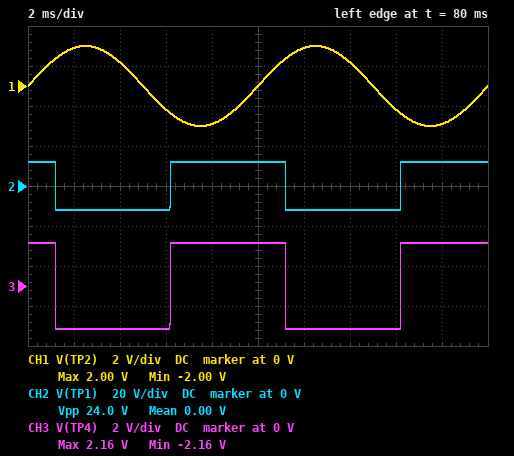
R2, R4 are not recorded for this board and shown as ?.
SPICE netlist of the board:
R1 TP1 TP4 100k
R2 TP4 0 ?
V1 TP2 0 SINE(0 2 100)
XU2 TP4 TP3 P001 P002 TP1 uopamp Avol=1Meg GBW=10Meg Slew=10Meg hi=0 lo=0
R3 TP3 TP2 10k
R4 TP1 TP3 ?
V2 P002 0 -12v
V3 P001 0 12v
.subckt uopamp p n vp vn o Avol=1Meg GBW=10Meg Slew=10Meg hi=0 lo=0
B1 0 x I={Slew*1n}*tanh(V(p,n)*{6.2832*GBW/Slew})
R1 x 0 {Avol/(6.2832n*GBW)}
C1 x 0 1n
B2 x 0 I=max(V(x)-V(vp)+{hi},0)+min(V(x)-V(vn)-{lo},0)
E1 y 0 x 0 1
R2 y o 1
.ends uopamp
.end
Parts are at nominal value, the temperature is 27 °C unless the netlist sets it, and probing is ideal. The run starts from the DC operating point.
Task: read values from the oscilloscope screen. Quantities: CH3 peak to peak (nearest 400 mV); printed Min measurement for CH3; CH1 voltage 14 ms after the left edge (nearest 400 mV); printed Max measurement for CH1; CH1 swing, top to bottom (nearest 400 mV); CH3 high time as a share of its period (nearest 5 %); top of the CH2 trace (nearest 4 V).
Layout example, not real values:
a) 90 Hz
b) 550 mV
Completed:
a) 4.4 V
b) -2.16 V
c) 1.2 V
d) 2.00 V
e) 4.0 V
f) 50 %
g) 12 V
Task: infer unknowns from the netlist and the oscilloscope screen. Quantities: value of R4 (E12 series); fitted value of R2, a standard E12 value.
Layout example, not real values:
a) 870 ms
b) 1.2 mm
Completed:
a) 120 kΩ
b) 22 kΩ
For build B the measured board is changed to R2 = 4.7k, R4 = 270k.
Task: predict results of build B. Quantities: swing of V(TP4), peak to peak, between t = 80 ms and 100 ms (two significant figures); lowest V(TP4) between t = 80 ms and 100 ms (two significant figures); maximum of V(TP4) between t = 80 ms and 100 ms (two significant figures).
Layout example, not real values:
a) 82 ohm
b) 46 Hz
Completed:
a) 1.1 V
b) -540 mV
c) 540 mV
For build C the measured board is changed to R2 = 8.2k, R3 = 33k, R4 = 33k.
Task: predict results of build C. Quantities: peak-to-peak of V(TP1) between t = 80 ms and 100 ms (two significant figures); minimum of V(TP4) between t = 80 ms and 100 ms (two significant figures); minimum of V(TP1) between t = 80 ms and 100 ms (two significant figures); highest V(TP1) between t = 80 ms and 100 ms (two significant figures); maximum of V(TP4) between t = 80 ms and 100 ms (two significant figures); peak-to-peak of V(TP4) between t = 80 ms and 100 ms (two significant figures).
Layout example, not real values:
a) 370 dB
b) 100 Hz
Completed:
a) 4.7 V
b) -180 mV
c) -2.4 V
d) 2.4 V
e) 180 mV
f) 360 mV
